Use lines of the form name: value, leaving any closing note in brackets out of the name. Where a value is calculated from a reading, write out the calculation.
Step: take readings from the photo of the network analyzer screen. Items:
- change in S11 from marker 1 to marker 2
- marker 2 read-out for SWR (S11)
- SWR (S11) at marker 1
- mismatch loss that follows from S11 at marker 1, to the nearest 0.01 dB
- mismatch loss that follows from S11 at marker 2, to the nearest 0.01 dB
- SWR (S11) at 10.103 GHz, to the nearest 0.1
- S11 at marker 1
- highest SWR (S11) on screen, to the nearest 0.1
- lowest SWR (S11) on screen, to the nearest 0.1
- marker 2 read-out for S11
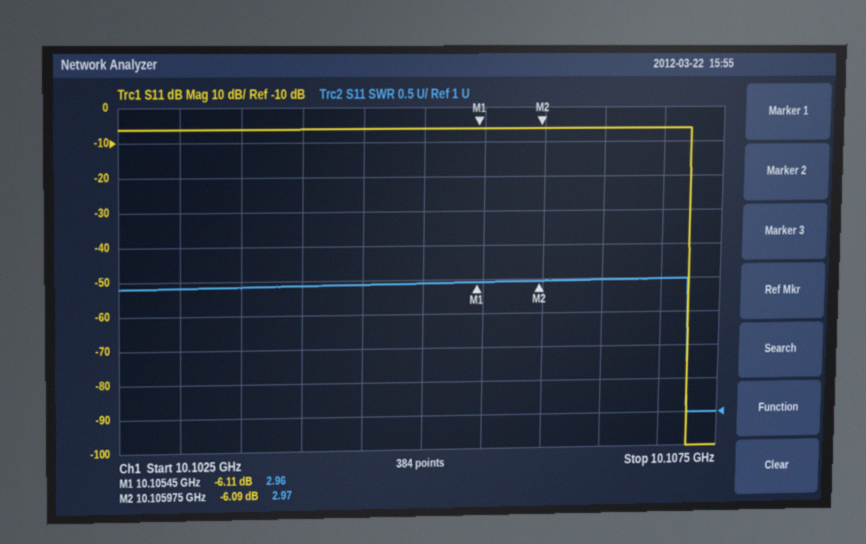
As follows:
change in S11 from marker 1 to marker 2: -6.09 − (-6.11) = 0.02 dB
marker 2 read-out for SWR: 2.97
SWR (S11) at marker 1: 2.96
mismatch loss that follows from S11 at marker 1, to the nearest 0.01 dB: −10 log10(1 − 10^(-6.11/10)) ≈ 1.22 dB
mismatch loss that follows from S11 at marker 2, to the nearest 0.01 dB: −10 log10(1 − 10^(-6.09/10)) ≈ 1.23 dB
SWR (S11) at 10.103 GHz, to the nearest 0.1: 2.9
S11 at marker 1: -6.11 dB
highest SWR (S11) on screen, to the nearest 0.1: 3.0
lowest SWR (S11) on screen, to the nearest 0.1: 1.0
marker 2 read-out for S11: -6.09 dB
